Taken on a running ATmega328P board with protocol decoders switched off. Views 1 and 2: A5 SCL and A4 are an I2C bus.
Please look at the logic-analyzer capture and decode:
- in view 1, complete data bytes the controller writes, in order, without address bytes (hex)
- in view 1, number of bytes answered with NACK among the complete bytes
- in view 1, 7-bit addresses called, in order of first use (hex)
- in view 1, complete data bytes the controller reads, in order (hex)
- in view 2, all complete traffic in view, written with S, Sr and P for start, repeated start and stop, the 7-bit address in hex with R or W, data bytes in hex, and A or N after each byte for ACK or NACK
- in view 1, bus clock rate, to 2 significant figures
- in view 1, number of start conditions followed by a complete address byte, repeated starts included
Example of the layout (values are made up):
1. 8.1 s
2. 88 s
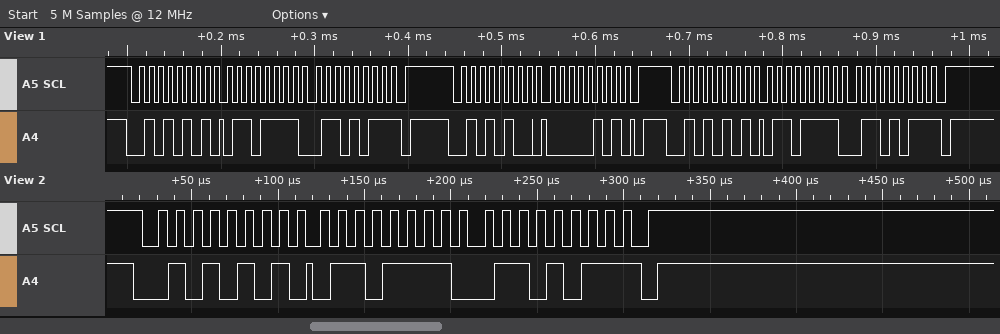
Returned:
1. 05
2. 2
3. 0x2A
4. 6F 6B 6F 6B
5. S 2AR A 6F A 6B N P
6. 100 kHz
7. 3
